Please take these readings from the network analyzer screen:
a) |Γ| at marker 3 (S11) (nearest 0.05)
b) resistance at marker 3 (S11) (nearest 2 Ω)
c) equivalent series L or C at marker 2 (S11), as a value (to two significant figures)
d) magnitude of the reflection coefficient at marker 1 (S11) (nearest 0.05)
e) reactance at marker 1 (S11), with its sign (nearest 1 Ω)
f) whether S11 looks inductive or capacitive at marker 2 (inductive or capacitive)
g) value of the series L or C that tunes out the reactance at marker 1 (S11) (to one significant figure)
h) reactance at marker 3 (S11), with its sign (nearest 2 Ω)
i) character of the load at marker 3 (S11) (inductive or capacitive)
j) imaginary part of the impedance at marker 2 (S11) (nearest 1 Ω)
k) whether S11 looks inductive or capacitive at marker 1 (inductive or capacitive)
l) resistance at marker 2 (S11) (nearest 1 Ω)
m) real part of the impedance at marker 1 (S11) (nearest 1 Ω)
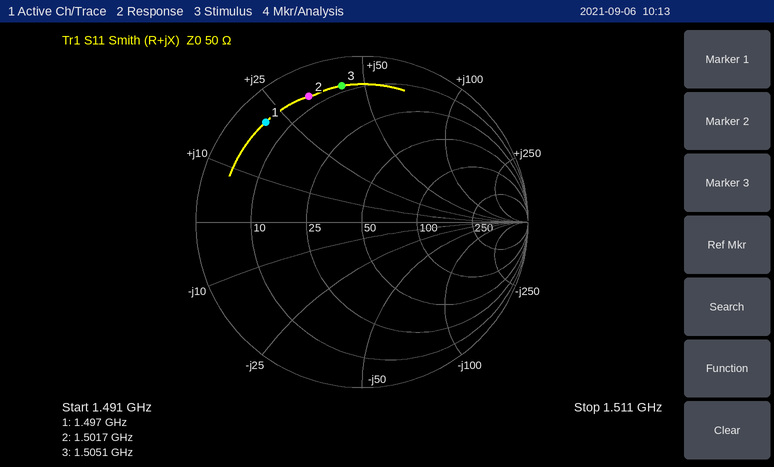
0.85
8 Ω
3.5 nH
0.85
+21 Ω
inductive
5 pF
+42 Ω
inductive
+33 Ω
inductive
7 Ω
5 Ω
